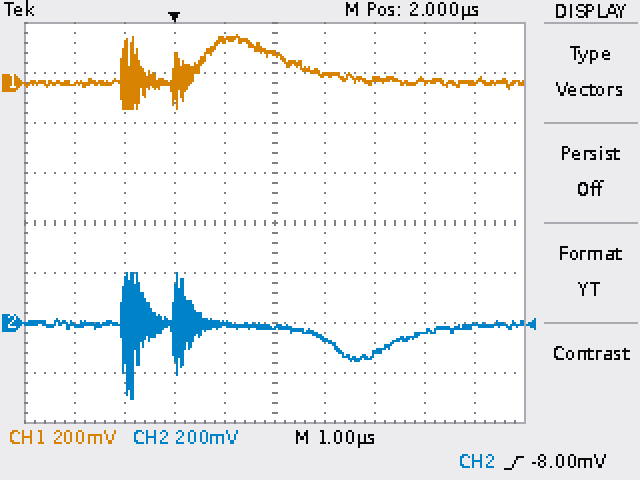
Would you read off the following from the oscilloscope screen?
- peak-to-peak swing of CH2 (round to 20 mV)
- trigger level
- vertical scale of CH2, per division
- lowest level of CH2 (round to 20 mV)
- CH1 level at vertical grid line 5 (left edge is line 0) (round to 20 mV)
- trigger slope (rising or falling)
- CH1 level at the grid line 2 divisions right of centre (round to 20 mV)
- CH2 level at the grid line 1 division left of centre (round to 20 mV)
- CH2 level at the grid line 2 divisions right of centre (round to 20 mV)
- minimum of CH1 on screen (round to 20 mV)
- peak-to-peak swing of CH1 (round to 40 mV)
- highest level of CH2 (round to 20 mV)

500 mV
-8.00 mV
200 mV
-300 mV
120 mV
rising
0 mV
0 mV
-120 mV
-100 mV
280 mV
200 mV
